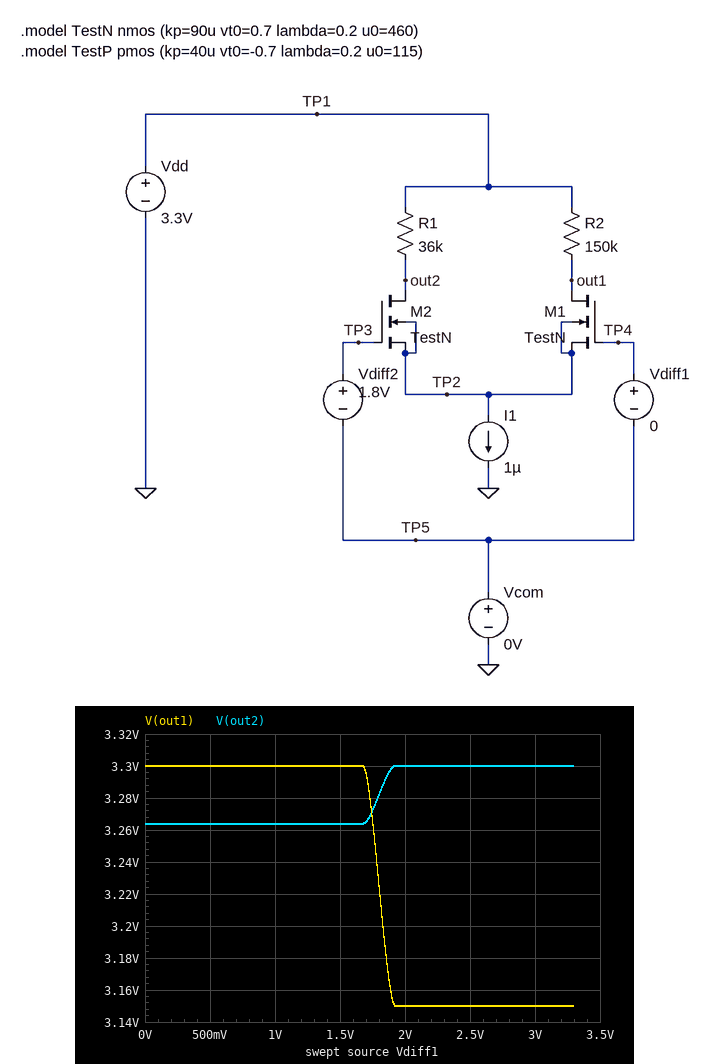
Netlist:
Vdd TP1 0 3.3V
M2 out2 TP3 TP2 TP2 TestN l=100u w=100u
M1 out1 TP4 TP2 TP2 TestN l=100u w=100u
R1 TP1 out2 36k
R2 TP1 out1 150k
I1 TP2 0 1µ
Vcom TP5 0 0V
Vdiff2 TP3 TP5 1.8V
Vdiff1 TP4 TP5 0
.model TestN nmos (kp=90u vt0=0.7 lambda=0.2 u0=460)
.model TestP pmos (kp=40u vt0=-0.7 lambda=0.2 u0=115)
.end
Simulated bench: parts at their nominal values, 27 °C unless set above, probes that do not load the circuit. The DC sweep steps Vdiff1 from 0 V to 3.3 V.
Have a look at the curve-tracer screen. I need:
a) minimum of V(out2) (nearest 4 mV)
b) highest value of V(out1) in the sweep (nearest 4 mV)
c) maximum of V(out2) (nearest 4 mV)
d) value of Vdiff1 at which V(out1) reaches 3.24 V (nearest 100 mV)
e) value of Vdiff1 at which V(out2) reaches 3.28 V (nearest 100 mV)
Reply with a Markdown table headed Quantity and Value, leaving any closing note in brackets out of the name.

| Quantity | Value |
|---|---|
| minimum of V(out2) | 3.264 V |
| highest value of V(out1) in the sweep | 3.300 V |
| maximum of V(out2) | 3.300 V |
| value of Vdiff1 at which V(out1) reaches 3.24 V | 1.8 V |
| value of Vdiff1 at which V(out2) reaches 3.28 V | 1.8 V |
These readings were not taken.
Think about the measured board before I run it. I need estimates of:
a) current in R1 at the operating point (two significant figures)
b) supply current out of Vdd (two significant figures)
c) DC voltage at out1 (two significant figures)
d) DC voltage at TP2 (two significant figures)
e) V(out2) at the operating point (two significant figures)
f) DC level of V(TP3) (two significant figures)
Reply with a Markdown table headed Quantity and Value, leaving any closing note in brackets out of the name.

| Quantity | Value |
|---|---|
| current in R1 at the operating point | 1.0 µA |
| supply current out of Vdd | 1.0 µA |
| DC voltage at out1 | 3.3 V |
| DC voltage at TP2 | 980 mV |
| V(out2) at the operating point | 3.3 V |
| DC level of V(TP3) | 1.8 V |
